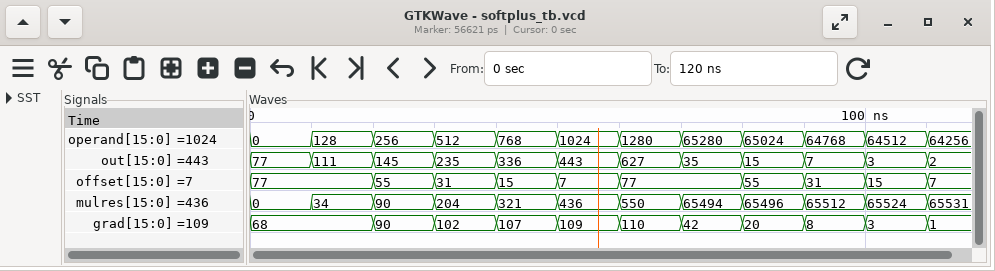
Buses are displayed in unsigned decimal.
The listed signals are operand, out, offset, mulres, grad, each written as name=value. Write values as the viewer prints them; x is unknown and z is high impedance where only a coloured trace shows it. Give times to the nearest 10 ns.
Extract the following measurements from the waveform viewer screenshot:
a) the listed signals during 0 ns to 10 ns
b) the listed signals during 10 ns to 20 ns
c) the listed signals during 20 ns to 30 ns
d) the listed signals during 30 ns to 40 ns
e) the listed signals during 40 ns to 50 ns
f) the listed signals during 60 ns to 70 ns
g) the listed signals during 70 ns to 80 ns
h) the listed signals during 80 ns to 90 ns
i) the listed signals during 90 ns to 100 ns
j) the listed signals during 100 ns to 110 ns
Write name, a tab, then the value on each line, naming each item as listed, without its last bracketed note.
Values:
the listed signals during 0 ns to 10 ns	operand=0, out=77, offset=77, mulres=0, grad=68
the listed signals during 10 ns to 20 ns	operand=128, out=111, offset=77, mulres=34, grad=68
the listed signals during 20 ns to 30 ns	operand=256, out=145, offset=55, mulres=90, grad=90
the listed signals during 30 ns to 40 ns	operand=512, out=235, offset=31, mulres=204, grad=102
the listed signals during 40 ns to 50 ns	operand=768, out=336, offset=15, mulres=321, grad=107
the listed signals during 60 ns to 70 ns	operand=1280, out=627, offset=77, mulres=550, grad=110
the listed signals during 70 ns to 80 ns	operand=65280, out=35, offset=77, mulres=65494, grad=42
the listed signals during 80 ns to 90 ns	operand=65024, out=15, offset=55, mulres=65496, grad=20
the listed signals during 90 ns to 100 ns	operand=64768, out=7, offset=31, mulres=65512, grad=8
the listed signals during 100 ns to 110 ns	operand=64512, out=3, offset=15, mulres=65524, grad=3
